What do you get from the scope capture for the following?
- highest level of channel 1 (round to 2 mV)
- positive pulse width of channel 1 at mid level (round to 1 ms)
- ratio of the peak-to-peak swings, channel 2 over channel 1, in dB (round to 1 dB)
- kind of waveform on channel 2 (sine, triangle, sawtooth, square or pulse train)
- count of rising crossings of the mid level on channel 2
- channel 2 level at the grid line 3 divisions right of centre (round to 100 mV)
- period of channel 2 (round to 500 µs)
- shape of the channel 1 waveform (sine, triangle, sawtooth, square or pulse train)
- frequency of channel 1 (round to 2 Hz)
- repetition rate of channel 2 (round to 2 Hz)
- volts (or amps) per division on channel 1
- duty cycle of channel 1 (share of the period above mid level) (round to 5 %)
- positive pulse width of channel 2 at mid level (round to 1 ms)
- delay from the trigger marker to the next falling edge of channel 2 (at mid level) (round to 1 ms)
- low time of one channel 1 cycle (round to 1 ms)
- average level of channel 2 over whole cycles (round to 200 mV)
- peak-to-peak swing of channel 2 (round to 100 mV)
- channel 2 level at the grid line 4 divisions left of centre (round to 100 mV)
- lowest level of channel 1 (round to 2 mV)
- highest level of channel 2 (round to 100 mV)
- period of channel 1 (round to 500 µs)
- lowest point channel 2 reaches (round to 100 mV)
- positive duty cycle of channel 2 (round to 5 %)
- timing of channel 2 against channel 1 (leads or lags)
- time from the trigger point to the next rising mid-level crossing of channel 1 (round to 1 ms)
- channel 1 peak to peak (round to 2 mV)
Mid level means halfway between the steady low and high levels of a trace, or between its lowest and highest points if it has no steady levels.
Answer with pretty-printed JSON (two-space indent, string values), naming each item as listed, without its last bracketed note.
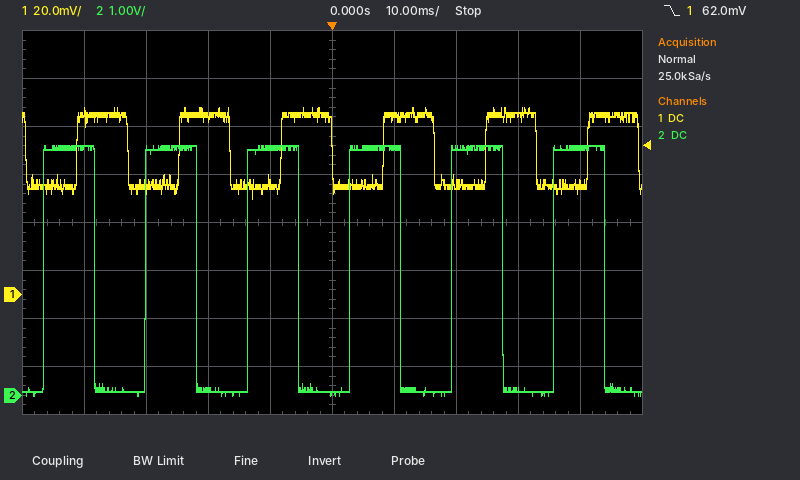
{
  "highest level of channel 1": "78 mV",
  "positive pulse width of channel 1 at mid level": "8 ms",
  "ratio of the peak-to-peak swings, channel 2 over channel 1, in dB": "43 dB",
  "kind of waveform on channel 2": "square",
  "count of rising crossings of the mid level on channel 2": "6",
  "channel 2 level at the grid line 3 divisions right of centre": "100 mV",
  "period of channel 2": "16.5 ms",
  "shape of the channel 1 waveform": "square",
  "frequency of channel 1": "60 Hz",
  "repetition rate of channel 2": "60 Hz",
  "volts (or amps) per division on channel 1": "20 mV",
  "duty cycle of channel 1 (share of the period above mid level)": "50 %",
  "positive pulse width of channel 2 at mid level": "8 ms",
  "delay from the trigger marker to the next falling edge of channel 2 (at mid level)": "11 ms",
  "low time of one channel 1 cycle": "8 ms",
  "average level of channel 2 over whole cycles": "2.6 V",
  "peak-to-peak swing of channel 2": "5.2 V",
  "channel 2 level at the grid line 4 divisions left of centre": "5.2 V",
  "lowest level of channel 1": "40 mV",
  "highest level of channel 2": "5.2 V",
  "period of channel 1": "16.5 ms",
  "lowest point channel 2 reaches": "0.0 V",
  "positive duty cycle of channel 2": "50 %",
  "timing of channel 2 against channel 1": "leads",
  "time from the trigger point to the next rising mid-level crossing of channel 1": "8 ms",
  "channel 1 peak to peak": "38 mV"
}
